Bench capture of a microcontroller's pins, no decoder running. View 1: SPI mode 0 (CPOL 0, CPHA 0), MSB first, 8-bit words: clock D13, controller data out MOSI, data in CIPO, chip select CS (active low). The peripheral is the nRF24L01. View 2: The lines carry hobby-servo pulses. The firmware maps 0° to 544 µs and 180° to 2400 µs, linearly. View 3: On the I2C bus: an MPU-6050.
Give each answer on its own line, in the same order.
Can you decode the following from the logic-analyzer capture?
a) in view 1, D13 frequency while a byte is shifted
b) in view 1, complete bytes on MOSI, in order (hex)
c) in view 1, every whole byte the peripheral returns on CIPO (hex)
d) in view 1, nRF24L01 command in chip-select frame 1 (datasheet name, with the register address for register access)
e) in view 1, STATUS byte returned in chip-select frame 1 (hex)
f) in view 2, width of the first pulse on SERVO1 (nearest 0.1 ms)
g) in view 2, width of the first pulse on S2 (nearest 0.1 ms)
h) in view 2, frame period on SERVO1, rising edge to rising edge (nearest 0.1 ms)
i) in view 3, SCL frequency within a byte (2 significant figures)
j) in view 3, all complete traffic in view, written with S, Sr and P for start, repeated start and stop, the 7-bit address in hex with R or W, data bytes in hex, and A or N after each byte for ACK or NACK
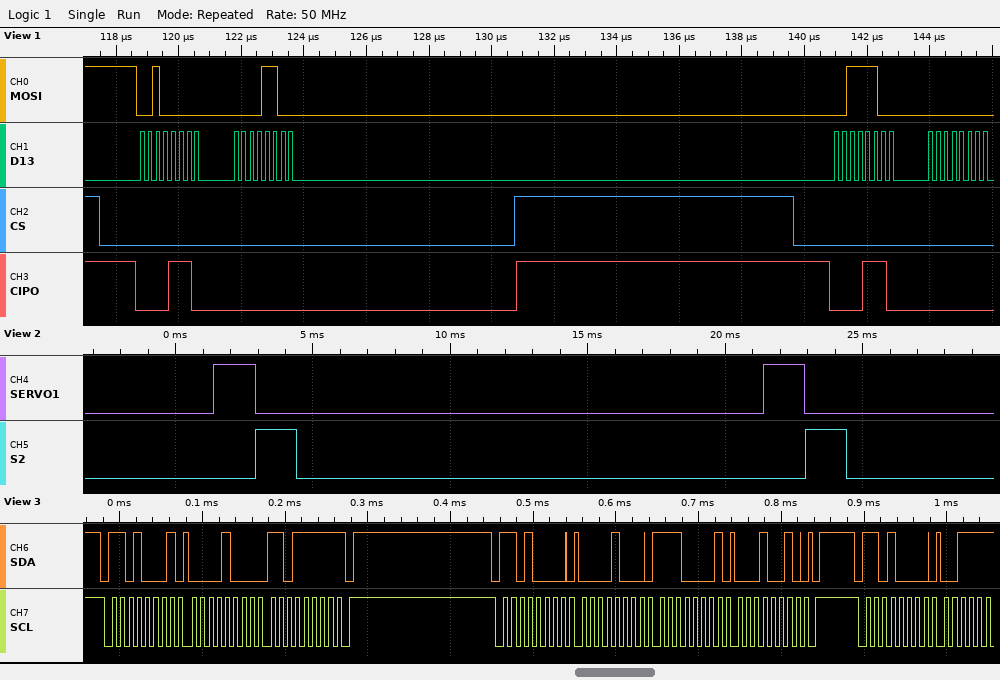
4 MHz
0x20 0x0C 0x3C 0x00
0x0E 0x00 0x0E 0x00
W_REGISTER 0x00
0x0E
1.5 ms
1.5 ms
20.0 ms
100 kHz
S 68R A 08 A DF N P S 68W A 08 A E1 A 12 A P S 68W A
